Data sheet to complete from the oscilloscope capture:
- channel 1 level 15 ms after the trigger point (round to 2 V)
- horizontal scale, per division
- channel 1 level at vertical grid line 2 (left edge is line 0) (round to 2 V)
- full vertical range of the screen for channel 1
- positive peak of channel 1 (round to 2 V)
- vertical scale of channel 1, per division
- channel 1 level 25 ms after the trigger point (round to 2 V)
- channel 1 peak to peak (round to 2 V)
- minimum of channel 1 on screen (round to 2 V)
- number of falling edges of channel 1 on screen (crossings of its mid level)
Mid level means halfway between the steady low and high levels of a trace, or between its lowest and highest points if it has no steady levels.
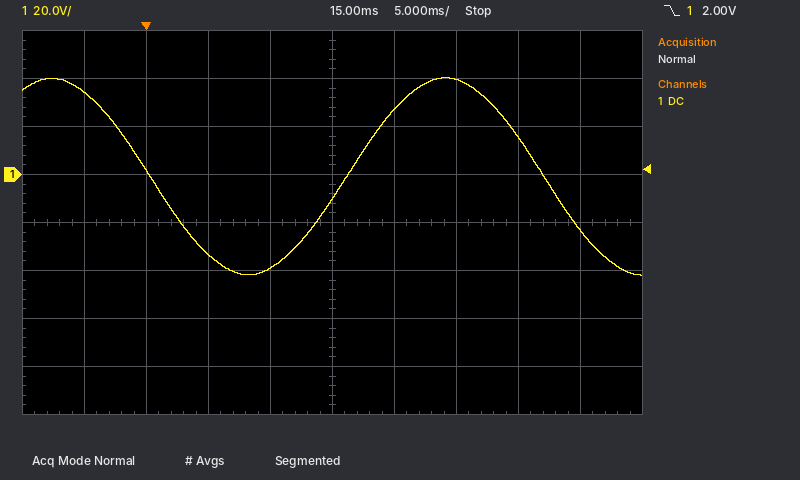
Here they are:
-10 V
5 ms
2 V
160 V
40 V
20 V
40 V
82 V
-42 V
2
